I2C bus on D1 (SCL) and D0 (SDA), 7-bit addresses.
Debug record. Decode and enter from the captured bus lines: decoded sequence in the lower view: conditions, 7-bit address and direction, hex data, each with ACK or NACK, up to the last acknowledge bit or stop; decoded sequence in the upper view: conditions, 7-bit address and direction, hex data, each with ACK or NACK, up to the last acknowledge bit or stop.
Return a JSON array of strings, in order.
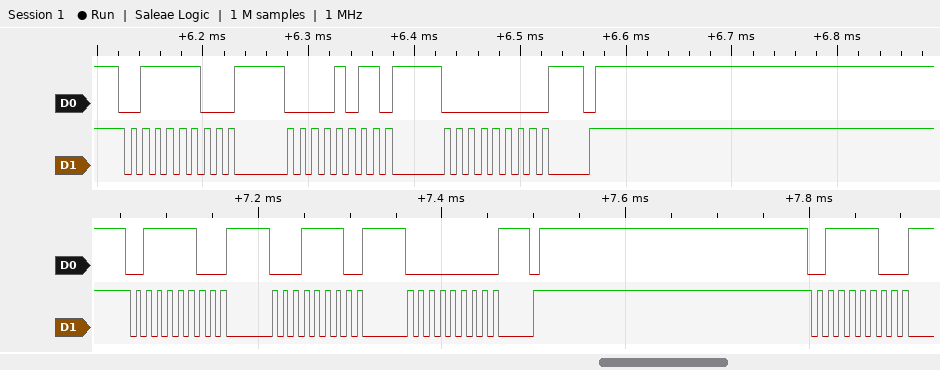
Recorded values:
["start, address 3E write ACK, 1E ACK, 00 ACK, stop, start, address 3E write ACK", "start, address 3E write ACK, 0B ACK, 00 ACK, stop"]
